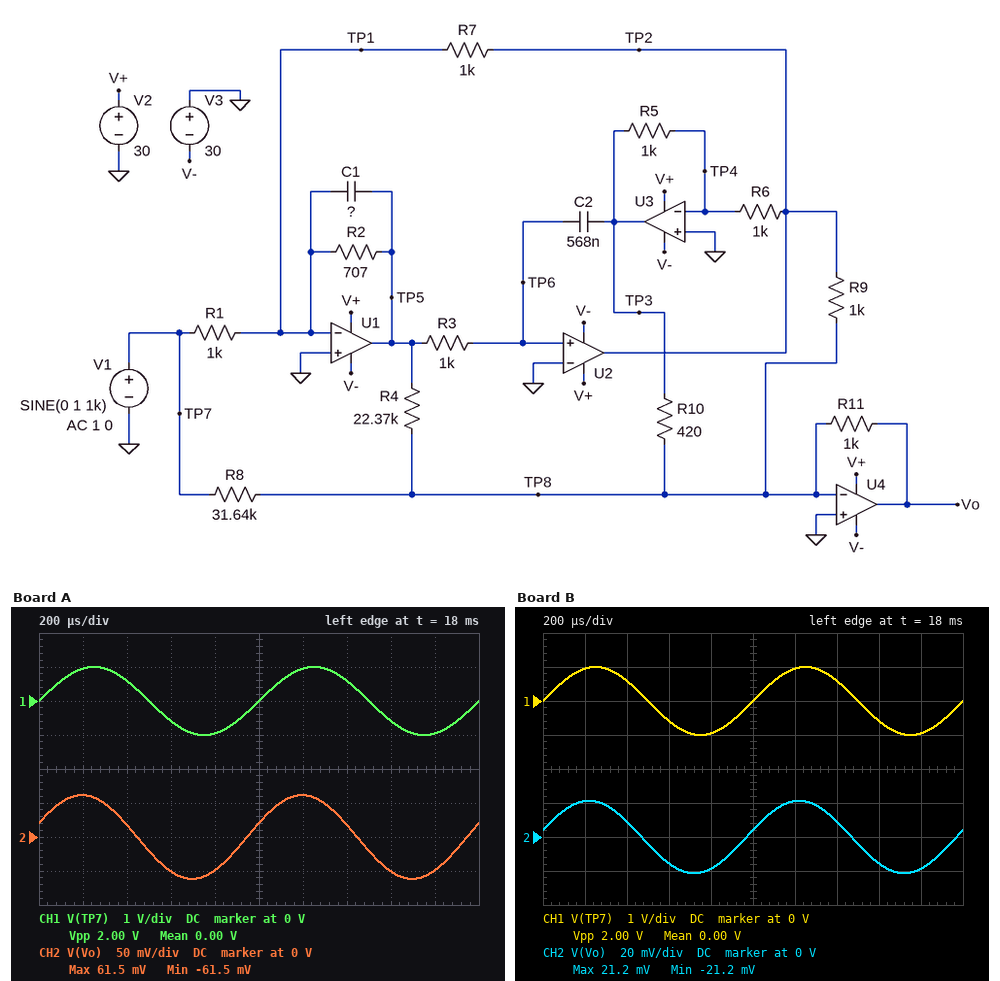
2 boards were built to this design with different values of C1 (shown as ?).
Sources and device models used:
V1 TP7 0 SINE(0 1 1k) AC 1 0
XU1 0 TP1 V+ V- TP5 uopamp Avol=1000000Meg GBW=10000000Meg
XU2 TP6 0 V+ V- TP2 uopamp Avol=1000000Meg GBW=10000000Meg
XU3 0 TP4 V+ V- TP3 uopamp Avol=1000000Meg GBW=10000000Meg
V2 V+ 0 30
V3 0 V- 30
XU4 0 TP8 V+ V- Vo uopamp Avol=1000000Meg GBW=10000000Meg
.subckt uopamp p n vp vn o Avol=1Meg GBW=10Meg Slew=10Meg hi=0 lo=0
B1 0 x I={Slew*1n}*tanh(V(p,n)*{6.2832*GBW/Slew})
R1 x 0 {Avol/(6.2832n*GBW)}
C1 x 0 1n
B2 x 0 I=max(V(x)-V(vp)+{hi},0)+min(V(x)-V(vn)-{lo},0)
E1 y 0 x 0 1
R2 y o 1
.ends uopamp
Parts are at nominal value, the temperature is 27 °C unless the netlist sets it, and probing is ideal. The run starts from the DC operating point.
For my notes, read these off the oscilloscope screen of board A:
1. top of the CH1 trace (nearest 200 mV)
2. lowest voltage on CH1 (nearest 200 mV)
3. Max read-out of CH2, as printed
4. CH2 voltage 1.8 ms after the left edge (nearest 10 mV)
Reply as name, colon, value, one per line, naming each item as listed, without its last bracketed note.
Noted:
top of the CH1 trace: 1.0 V
lowest voltage on CH1: -1.0 V
Max read-out of CH2, as printed: 61.5 mV
CH2 voltage 1.8 ms after the left edge: -50 mV
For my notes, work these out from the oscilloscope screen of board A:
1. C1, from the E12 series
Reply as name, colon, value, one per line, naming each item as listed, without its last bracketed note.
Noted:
C1, from the E12 series: 680 nF
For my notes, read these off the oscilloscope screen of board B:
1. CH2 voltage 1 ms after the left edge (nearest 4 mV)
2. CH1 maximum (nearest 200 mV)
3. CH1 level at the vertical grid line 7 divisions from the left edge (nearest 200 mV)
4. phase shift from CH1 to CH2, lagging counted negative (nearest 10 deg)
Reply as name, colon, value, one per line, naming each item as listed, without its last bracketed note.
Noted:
CH2 voltage 1 ms after the left edge: 4 mV
CH1 maximum: 1.0 V
CH1 level at the vertical grid line 7 divisions from the left edge: 600 mV
phase shift from CH1 to CH2, lagging counted negative: 10 deg
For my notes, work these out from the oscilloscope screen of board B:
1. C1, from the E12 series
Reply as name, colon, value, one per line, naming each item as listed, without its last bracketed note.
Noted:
C1, from the E12 series: 1.2 µF
